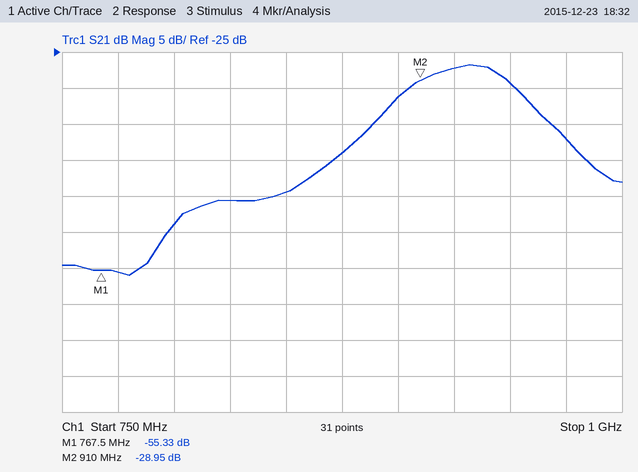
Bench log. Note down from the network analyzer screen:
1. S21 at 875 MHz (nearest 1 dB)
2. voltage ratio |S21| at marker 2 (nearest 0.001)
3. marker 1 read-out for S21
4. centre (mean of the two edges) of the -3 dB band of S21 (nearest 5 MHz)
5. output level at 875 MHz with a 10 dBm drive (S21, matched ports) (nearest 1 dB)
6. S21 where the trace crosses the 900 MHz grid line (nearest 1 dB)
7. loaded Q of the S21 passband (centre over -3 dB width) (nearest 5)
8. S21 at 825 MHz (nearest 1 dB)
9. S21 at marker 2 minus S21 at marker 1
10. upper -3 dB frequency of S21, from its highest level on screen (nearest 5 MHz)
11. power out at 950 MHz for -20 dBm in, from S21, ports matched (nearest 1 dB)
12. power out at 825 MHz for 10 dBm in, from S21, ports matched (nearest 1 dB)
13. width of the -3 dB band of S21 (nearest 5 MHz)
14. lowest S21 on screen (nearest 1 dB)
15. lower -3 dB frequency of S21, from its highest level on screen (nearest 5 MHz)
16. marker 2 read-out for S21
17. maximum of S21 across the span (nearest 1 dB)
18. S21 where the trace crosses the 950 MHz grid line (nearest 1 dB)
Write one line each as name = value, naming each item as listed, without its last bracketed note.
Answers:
S21 at 875 MHz = -39 dB
voltage ratio |S21| at marker 2 = 0.036
marker 1 read-out for S21 = -55.33 dB
centre (mean of the two edges) of the -3 dB band of S21 = 930 MHz
output level at 875 MHz with a 10 dBm drive (S21, matched ports) = -29 dBm
S21 where the trace crosses the 900 MHz grid line = -31 dB
loaded Q of the S21 passband (centre over -3 dB width) = 20
S21 at 825 MHz = -46 dB
S21 at marker 2 minus S21 at marker 1 = 26.38 dB
upper -3 dB frequency of S21, from its highest level on screen = 950 MHz
power out at 950 MHz for -20 dBm in, from S21, ports matched = -49 dBm
power out at 825 MHz for 10 dBm in, from S21, ports matched = -36 dBm
width of the -3 dB band of S21 = 45 MHz
lowest S21 on screen = -56 dB
lower -3 dB frequency of S21, from its highest level on screen = 905 MHz
marker 2 read-out for S21 = -28.95 dB
maximum of S21 across the span = -27 dB
S21 where the trace crosses the 950 MHz grid line = -29 dB
